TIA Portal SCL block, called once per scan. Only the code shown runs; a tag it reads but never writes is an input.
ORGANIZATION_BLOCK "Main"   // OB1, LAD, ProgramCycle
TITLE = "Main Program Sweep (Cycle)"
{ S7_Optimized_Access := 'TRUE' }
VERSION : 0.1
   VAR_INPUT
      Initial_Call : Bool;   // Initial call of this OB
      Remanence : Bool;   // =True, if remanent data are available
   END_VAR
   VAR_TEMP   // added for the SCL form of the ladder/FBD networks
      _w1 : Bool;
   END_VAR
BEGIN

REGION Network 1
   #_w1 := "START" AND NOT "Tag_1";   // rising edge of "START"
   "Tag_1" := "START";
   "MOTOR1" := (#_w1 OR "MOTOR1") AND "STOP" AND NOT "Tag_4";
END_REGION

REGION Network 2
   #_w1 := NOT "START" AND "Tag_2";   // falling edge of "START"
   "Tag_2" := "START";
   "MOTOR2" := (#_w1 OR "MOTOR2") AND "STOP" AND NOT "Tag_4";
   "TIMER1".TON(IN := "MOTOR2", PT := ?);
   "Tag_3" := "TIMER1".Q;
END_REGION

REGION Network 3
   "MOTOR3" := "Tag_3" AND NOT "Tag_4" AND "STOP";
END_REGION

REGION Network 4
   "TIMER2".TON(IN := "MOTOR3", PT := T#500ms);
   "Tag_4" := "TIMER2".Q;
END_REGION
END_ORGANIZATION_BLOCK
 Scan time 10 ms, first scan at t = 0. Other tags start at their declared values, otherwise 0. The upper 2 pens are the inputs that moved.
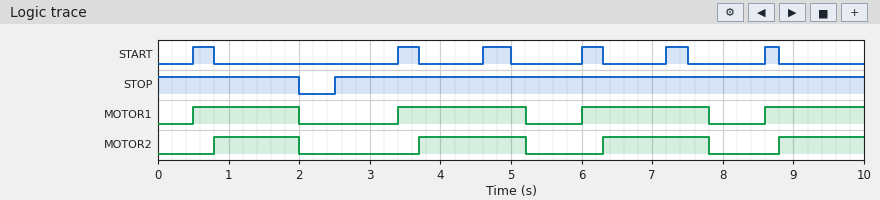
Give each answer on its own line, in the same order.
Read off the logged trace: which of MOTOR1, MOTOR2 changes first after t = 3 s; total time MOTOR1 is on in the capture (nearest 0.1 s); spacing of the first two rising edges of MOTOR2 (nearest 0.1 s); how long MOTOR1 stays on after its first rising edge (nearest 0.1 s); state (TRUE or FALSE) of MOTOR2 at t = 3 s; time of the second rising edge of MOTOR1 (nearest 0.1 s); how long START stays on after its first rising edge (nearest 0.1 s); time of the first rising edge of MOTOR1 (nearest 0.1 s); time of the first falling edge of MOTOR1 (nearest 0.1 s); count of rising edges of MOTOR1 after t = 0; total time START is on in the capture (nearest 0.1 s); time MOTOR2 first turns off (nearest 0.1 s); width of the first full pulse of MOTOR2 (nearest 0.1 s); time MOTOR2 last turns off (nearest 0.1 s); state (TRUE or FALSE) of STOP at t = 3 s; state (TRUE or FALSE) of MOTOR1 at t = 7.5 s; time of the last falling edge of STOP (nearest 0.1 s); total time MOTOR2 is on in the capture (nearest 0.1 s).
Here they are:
MOTOR1
6.5 s
2.9 s
1.5 s
FALSE
3.4 s
0.3 s
0.5 s
2.0 s
4
1.8 s
2.0 s
1.2 s
7.8 s
TRUE
TRUE
2.0 s
5.4 s
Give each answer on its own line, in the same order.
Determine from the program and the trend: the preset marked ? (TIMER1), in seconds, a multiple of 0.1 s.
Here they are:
1.0 s
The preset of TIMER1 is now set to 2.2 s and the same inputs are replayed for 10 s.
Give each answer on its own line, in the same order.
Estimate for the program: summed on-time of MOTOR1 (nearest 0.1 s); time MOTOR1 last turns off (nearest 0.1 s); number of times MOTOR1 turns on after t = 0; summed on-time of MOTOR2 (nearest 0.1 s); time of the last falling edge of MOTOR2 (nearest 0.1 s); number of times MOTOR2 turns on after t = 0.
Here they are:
7.3 s
6.4 s
3
6.4 s
6.4 s
3
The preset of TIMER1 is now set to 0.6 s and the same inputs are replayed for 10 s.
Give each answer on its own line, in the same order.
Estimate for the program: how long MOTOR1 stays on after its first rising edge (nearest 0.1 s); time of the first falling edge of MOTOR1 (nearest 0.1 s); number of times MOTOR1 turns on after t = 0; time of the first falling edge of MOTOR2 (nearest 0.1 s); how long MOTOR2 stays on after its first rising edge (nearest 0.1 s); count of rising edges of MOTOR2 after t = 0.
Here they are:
1.4 s
1.9 s
5
1.9 s
1.1 s
6
